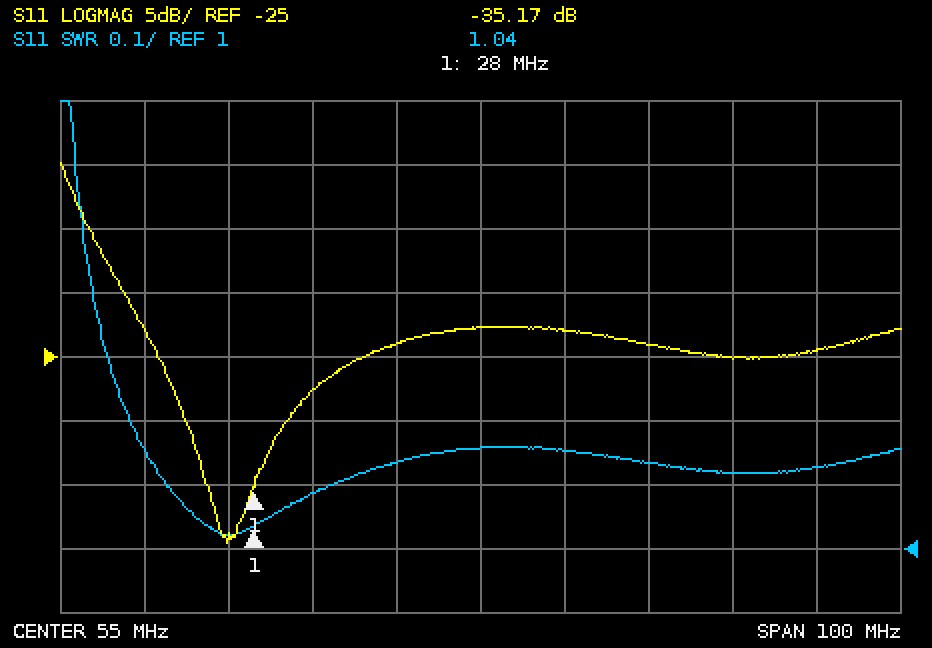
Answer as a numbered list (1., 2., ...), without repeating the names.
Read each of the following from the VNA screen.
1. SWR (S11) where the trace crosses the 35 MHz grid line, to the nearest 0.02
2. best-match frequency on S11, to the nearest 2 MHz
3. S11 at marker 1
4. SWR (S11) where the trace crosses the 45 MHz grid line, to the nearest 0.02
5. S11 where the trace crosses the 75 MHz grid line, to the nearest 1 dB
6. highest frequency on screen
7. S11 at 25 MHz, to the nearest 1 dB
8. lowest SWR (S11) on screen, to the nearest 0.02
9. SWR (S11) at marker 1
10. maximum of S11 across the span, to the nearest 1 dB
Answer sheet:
1. 1.08
2. 24 MHz
3. -35.17 dB
4. 1.14
5. -24 dB
6. 105 MHz
7. -39 dB
8. 1.02
9. 1.04
10. -10 dB
